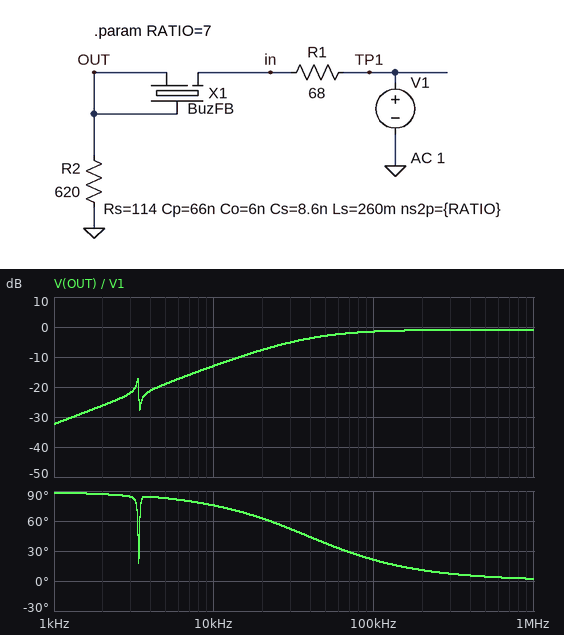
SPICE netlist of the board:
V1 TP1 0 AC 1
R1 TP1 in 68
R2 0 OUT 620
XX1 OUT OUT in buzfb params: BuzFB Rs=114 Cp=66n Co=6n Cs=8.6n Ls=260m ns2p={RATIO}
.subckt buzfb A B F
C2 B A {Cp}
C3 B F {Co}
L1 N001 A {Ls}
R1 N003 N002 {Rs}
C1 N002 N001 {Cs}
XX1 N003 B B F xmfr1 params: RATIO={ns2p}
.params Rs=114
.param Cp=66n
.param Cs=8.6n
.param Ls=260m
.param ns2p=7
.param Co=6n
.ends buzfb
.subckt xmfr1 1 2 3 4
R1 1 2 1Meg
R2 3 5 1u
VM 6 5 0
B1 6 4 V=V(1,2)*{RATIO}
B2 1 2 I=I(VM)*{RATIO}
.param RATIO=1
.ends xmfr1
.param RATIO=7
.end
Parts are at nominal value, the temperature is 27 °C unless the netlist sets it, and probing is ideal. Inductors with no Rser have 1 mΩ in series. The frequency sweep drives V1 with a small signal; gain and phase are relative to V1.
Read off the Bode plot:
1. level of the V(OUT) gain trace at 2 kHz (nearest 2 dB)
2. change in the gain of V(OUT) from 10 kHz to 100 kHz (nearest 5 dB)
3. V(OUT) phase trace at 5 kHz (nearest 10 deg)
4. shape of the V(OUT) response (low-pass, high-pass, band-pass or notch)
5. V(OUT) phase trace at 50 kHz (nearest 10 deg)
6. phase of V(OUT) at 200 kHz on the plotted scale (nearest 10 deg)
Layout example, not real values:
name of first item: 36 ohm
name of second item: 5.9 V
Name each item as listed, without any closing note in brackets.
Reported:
level of the V(OUT) gain trace at 2 kHz: -26 dB
change in the gain of V(OUT) from 10 kHz to 100 kHz: 10 dB
V(OUT) phase trace at 5 kHz: 80 deg
shape of the V(OUT) response: high-pass
V(OUT) phase trace at 50 kHz: 40 deg
phase of V(OUT) at 200 kHz on the plotted scale: 10 deg
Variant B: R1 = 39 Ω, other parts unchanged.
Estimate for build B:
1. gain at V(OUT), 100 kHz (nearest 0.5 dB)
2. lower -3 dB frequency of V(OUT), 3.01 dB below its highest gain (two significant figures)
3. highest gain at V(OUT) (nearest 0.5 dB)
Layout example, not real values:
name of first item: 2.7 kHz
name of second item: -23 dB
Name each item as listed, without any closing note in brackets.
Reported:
gain at V(OUT), 100 kHz: -1.0 dB
lower -3 dB frequency of V(OUT), 3.01 dB below its highest gain: 40 kHz
highest gain at V(OUT): -0.5 dB
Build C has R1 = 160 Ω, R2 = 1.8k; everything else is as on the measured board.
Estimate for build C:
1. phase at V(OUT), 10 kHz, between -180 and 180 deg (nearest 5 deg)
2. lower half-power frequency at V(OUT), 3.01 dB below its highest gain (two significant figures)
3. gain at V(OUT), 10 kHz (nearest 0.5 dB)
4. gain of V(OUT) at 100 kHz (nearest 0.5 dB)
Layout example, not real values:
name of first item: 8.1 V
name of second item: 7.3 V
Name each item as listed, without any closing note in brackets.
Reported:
phase at V(OUT), 10 kHz, between -180 and 180 deg: 55 deg
lower half-power frequency at V(OUT), 3.01 dB below its highest gain: 14 kHz
gain at V(OUT), 10 kHz: -5.5 dB
gain of V(OUT) at 100 kHz: -1.0 dB
